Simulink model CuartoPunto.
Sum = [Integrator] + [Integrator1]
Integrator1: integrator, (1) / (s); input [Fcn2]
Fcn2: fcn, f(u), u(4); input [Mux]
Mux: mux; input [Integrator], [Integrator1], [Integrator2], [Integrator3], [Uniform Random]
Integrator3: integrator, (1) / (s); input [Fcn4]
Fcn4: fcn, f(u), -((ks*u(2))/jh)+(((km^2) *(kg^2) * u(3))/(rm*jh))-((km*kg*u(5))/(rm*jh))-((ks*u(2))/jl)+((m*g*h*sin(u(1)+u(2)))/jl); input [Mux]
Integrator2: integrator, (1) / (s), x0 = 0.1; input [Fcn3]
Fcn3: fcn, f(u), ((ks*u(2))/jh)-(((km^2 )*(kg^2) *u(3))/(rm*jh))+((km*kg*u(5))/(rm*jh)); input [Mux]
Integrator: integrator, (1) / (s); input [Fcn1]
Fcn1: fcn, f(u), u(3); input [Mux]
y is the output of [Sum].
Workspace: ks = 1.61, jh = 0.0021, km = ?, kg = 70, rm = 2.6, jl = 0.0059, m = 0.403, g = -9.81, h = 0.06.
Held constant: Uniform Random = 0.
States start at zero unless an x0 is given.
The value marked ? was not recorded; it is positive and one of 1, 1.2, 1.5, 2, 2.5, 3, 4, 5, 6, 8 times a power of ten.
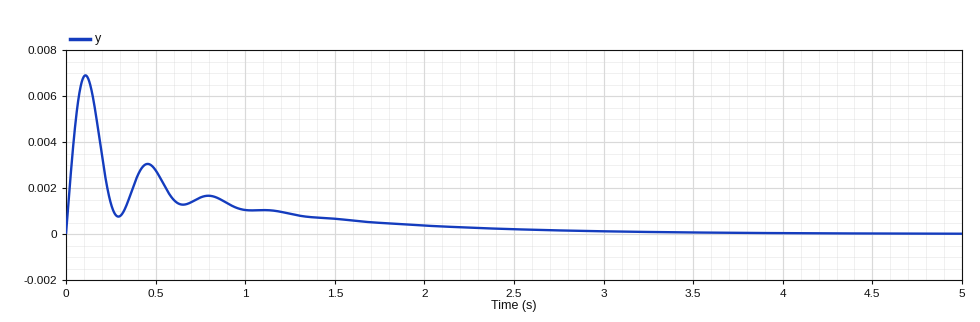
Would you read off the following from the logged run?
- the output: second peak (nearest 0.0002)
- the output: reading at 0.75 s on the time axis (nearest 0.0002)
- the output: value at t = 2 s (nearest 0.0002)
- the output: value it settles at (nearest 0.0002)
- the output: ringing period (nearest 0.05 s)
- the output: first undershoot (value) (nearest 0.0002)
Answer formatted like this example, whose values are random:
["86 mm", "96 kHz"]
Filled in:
["0.0030", "0.0016", "0.0004", "0.0000", "0.35 s", "0.0008"]
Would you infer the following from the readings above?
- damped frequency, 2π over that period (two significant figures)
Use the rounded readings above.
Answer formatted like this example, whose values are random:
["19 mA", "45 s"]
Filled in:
["18 rad/s"]
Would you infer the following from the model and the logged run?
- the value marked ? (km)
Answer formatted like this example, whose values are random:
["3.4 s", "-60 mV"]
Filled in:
["0.01"]
